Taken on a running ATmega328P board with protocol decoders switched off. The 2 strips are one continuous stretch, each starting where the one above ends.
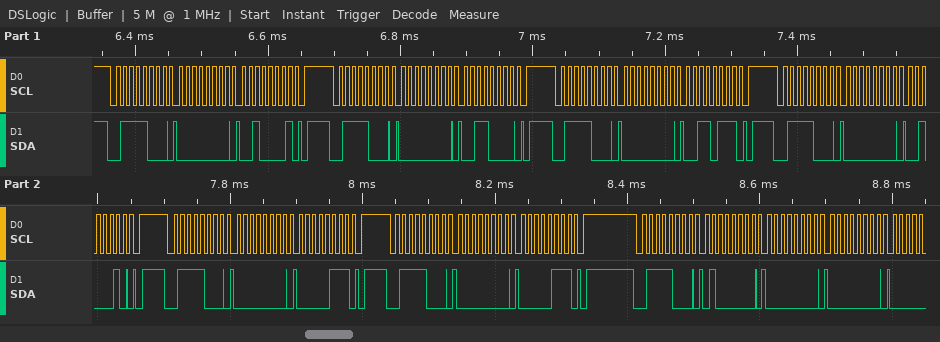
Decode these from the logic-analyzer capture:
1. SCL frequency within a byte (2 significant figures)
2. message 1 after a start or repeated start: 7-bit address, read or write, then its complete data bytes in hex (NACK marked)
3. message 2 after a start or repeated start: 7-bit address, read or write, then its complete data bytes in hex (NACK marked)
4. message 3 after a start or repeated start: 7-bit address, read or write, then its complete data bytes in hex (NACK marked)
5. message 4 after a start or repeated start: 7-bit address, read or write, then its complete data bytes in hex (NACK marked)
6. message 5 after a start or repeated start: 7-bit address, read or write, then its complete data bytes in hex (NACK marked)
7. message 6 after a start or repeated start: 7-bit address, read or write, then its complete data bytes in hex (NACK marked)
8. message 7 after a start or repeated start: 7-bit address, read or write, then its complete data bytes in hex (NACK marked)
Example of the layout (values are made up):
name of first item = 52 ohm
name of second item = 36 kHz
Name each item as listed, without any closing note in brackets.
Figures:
SCL frequency within a byte = 100 kHz
message 1 after a start or repeated start: 7-bit address, read or write, then its complete data bytes in hex = 0x3C write: 00 21
message 2 after a start or repeated start: 7-bit address, read or write, then its complete data bytes in hex = 0x3C write: 00 30
message 3 after a start or repeated start: 7-bit address, read or write, then its complete data bytes in hex = 0x3C write: 00 37
message 4 after a start or repeated start: 7-bit address, read or write, then its complete data bytes in hex = 0x3C write: 00 22
message 5 after a start or repeated start: 7-bit address, read or write, then its complete data bytes in hex = 0x3C write: 00 07
message 6 after a start or repeated start: 7-bit address, read or write, then its complete data bytes in hex = 0x3C write: 00 07
message 7 after a start or repeated start: 7-bit address, read or write, then its complete data bytes in hex = 0x3C write: 40 00 00
